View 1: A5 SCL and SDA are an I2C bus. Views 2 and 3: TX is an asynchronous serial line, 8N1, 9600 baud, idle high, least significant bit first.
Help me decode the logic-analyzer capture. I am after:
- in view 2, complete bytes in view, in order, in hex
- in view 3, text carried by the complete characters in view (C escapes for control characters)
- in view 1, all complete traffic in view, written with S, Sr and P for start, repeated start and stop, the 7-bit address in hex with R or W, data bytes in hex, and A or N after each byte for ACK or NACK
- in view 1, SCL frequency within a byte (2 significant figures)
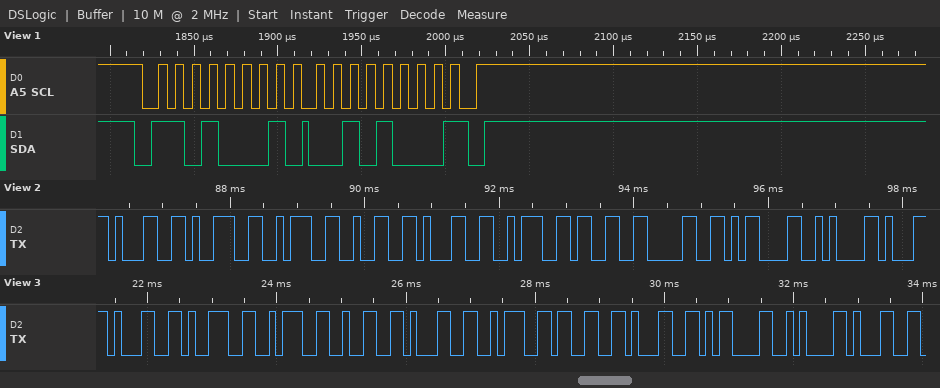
31 39 3A 32 31 3A 33 30 0D 0A
"19:21:31\r\n1"
S 68R A 28 N P
100 kHz
